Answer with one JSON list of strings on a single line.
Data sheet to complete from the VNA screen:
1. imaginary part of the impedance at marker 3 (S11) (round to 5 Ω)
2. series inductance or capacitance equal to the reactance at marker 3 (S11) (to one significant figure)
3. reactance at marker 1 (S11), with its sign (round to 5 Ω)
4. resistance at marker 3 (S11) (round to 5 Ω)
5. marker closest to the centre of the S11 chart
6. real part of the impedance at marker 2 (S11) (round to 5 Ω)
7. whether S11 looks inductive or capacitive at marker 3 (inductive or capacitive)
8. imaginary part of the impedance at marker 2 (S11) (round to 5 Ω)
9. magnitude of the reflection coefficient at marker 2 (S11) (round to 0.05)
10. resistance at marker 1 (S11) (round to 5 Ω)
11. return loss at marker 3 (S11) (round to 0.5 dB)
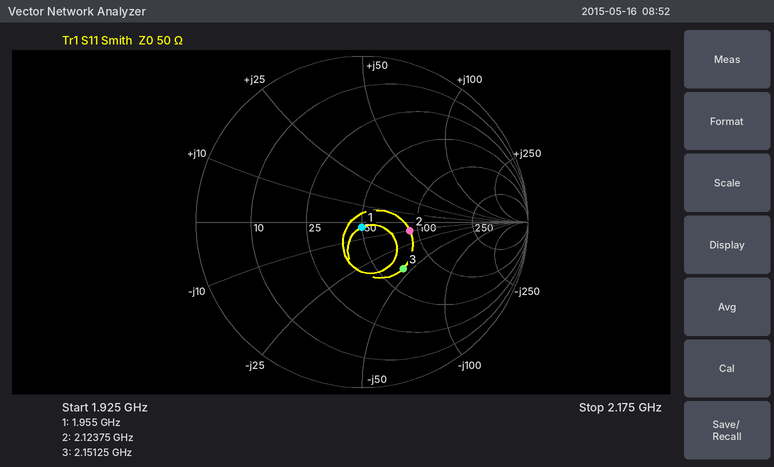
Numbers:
["-45 Ω", "2 pF", "-5 Ω", "65 Ω", "marker 1", "90 Ω", "capacitive", "-10 Ω", "0.30", "50 Ω", "8.5 dB"]
